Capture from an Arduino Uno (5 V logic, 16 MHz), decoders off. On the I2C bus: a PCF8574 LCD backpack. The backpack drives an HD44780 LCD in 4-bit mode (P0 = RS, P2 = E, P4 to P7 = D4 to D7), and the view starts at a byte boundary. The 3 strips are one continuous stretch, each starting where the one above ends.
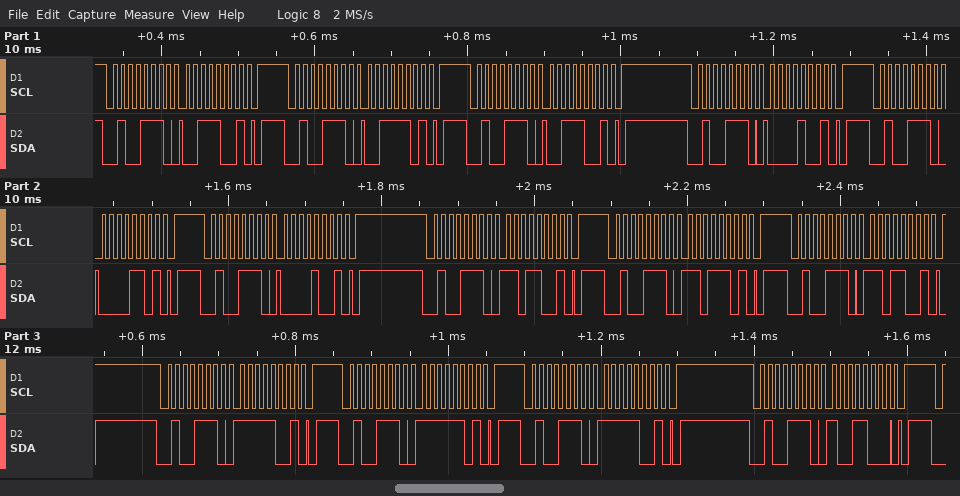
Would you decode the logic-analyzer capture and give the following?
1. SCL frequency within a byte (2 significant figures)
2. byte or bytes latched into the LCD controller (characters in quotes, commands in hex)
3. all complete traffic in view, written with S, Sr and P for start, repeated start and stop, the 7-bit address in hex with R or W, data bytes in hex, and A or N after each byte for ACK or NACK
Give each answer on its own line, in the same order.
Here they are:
100 kHz
'0' data 0xDF
S 27W A 39 A P S 27W A 3D A P S 27W A 39 A P S 27W A 09 A P S 27W A 0D A P S 27W A 09 A P S 27W A D9 A P S 27W A DD A P S 27W A D9 A P S 27W A F9 A P S 27W A FD A P S 27W A F9 A P S 27W A 98 A P
